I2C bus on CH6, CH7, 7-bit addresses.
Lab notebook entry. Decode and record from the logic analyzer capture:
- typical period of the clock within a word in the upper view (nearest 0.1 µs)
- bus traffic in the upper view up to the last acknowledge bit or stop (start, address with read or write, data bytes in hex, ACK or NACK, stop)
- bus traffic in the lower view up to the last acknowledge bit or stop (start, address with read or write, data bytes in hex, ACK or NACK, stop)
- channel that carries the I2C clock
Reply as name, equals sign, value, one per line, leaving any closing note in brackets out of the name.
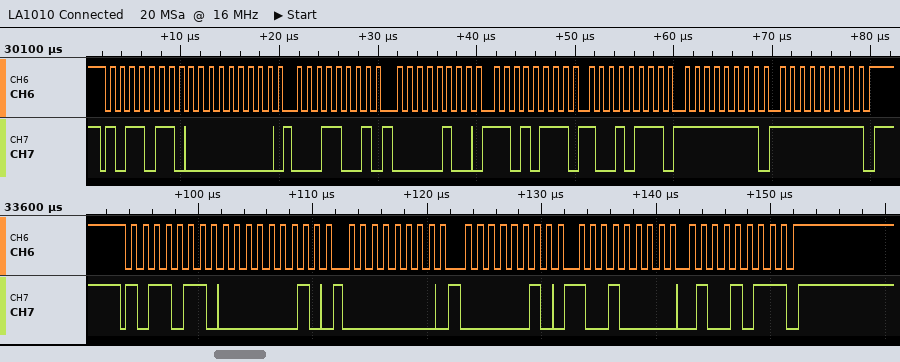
typical period of the clock within a word in the upper view = 1 µs
bus traffic in the upper view up to the last acknowledge bit or stop = start, address 5B write ACK, 00 ACK, 19 ACK, 04 ACK, D7 ACK, 97 ACK, FF ACK, FF NACK, stop
bus traffic in the lower view up to the last acknowledge bit or stop = start, address 5B write ACK, 02 ACK, 00 ACK, 02 ACK, 90 ACK, 4B NACK, stop
channel that carries the I2C clock = CH6
